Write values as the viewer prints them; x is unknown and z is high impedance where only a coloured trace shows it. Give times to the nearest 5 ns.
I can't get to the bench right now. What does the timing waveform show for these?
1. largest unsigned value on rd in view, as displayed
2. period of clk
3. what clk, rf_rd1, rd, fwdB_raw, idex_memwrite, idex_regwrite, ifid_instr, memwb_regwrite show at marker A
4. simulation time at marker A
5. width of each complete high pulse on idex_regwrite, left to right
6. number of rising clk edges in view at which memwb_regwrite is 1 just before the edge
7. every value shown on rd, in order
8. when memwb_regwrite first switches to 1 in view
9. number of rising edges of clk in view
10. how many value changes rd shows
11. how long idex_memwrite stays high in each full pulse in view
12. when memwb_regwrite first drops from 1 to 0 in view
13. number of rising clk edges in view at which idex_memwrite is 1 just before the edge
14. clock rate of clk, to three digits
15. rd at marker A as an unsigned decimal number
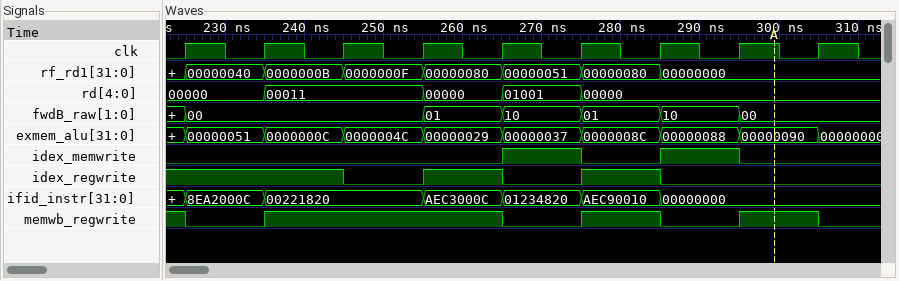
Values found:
01001
10 ns
clk=1, rf_rd1=00000000, rd=00000, fwdB_raw=00, idex_memwrite=0, idex_regwrite=0, ifid_instr=00000000, memwb_regwrite=1
300 ns
10 ns, 10 ns
6
00000, 00011, 00000, 01001, 00000
235 ns
9
4
10 ns, 10 ns
225 ns
2
100 MHz
0
